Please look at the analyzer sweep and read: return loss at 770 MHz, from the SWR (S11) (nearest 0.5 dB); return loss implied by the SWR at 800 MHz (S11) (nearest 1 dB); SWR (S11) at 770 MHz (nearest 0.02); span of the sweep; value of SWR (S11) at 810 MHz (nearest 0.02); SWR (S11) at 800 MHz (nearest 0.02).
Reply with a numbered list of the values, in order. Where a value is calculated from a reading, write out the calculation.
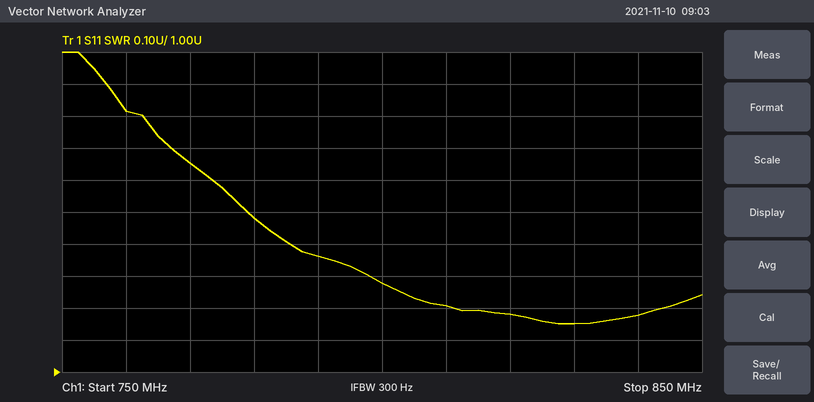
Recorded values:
1. −20 log10((1.66 − 1)/(1.66 + 1)) ≈ 12.1 dB, so 12.0 dB to the nearest 0.5 dB
2. −20 log10((1.28 − 1)/(1.28 + 1)) ≈ 18 dB
3. 1.66
4. 100 MHz
5. 1.20
6. 1.28
